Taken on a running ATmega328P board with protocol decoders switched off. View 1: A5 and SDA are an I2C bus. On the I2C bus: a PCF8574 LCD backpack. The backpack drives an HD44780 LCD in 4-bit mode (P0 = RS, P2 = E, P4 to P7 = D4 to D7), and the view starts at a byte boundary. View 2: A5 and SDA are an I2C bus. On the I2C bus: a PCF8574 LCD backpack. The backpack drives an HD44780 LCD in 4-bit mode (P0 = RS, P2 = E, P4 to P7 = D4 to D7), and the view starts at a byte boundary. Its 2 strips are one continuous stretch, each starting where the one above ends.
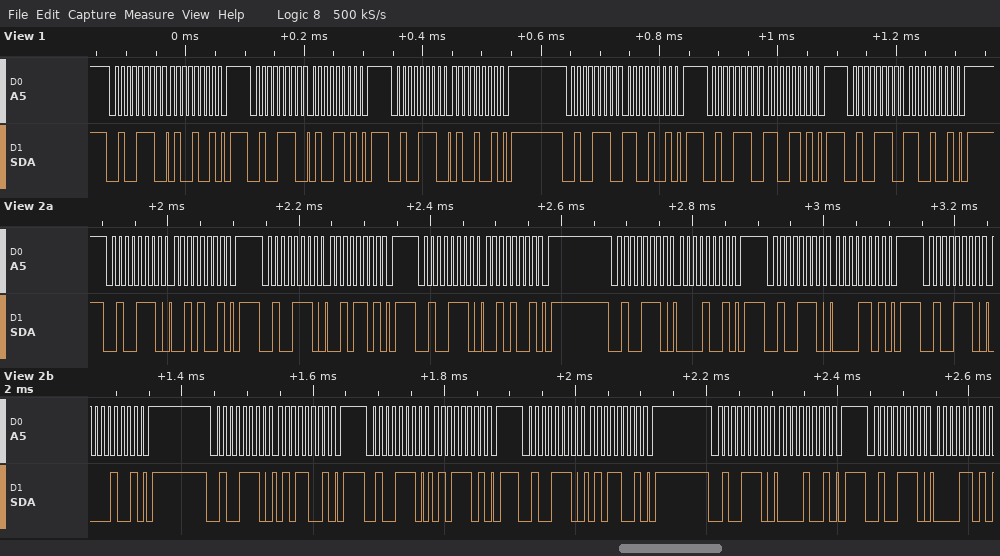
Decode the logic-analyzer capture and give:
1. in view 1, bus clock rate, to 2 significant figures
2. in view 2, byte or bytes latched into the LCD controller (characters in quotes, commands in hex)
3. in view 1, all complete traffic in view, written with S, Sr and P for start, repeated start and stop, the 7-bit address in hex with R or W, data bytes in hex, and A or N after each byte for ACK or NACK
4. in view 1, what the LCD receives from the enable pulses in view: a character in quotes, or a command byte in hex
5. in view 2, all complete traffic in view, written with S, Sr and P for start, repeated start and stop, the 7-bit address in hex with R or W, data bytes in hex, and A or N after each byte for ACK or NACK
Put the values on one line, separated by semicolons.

100 kHz; ' '; S 27W A 49 A P S 27W A 4D A P S 27W A 49 A P S 27W A C9 A P S 27W A CD A P S 27W A C9 A P; 'L'; S 27W A 29 A P S 27W A 2D A P S 27W A 29 A P S 27W A 09 A P S 27W A 0D A P S 27W A 09 A P S 27W A 59 A P S 27W A 5D A P S 27W A 59 A P S 27W A 09 A P S 27W A 0D A
